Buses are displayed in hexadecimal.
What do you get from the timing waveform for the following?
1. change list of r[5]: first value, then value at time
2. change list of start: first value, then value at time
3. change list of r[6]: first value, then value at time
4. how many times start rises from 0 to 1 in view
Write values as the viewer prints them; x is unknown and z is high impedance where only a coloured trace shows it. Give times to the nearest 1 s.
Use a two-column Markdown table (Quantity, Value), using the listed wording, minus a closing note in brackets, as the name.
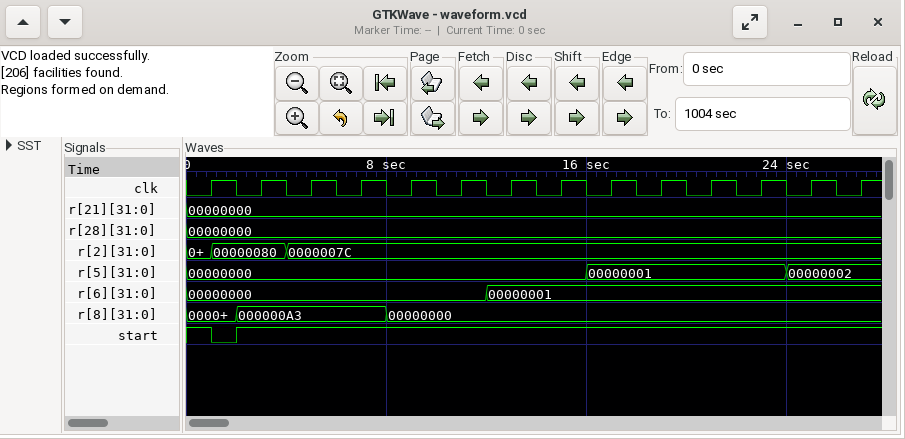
| Quantity | Value |
|---|---|
| change list of r[5]: first value, then value at time | 00000000, 00000001 at 16 s, 00000002 at 24 s |
| change list of start: first value, then value at time | 1, 0 at 1 s, 1 at 2 s |
| change list of r[6]: first value, then value at time | 00000000, 00000001 at 12 s |
| how many times start rises from 0 to 1 in view | 1 |
